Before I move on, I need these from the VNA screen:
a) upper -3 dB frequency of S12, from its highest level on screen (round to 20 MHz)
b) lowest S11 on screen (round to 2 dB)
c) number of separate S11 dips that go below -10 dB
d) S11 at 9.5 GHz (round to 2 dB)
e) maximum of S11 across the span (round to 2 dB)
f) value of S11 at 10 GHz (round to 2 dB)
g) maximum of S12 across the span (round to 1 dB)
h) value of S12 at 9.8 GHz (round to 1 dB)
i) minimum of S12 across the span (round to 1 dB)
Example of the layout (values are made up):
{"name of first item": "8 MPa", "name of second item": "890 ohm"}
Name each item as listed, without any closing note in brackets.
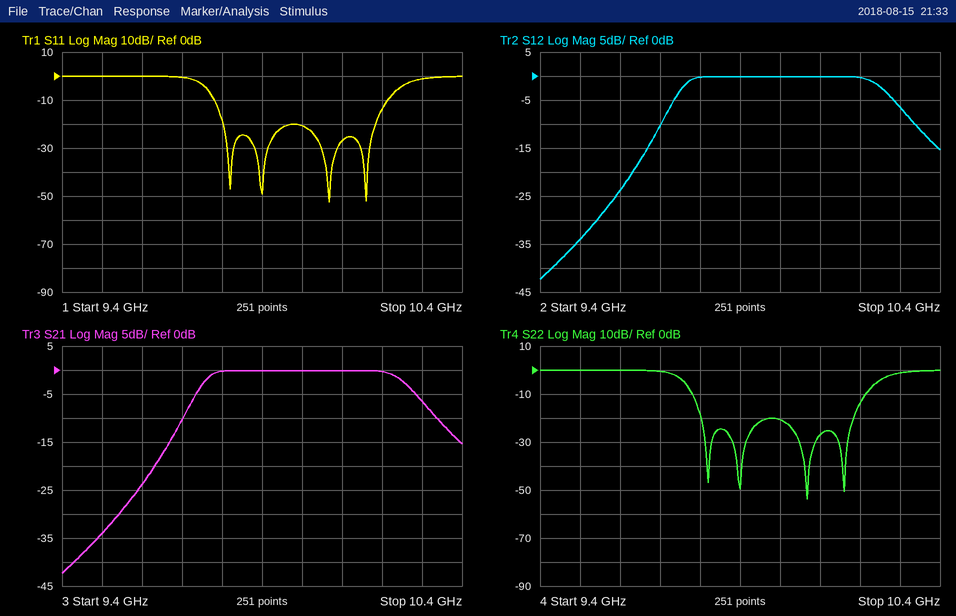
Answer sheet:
{"upper -3 dB frequency of S12, from its highest level on screen": "10.26 GHz", "lowest S11 on screen": "-52 dB", "number of separate S11 dips that go below -10 dB": "4", "S11 at 9.5 GHz": "0 dB", "maximum of S11 across the span": "0 dB", "value of S11 at 10 GHz": "-20 dB", "maximum of S12 across the span": "0 dB", "value of S12 at 9.8 GHz": "0 dB", "minimum of S12 across the span": "-42 dB"}
